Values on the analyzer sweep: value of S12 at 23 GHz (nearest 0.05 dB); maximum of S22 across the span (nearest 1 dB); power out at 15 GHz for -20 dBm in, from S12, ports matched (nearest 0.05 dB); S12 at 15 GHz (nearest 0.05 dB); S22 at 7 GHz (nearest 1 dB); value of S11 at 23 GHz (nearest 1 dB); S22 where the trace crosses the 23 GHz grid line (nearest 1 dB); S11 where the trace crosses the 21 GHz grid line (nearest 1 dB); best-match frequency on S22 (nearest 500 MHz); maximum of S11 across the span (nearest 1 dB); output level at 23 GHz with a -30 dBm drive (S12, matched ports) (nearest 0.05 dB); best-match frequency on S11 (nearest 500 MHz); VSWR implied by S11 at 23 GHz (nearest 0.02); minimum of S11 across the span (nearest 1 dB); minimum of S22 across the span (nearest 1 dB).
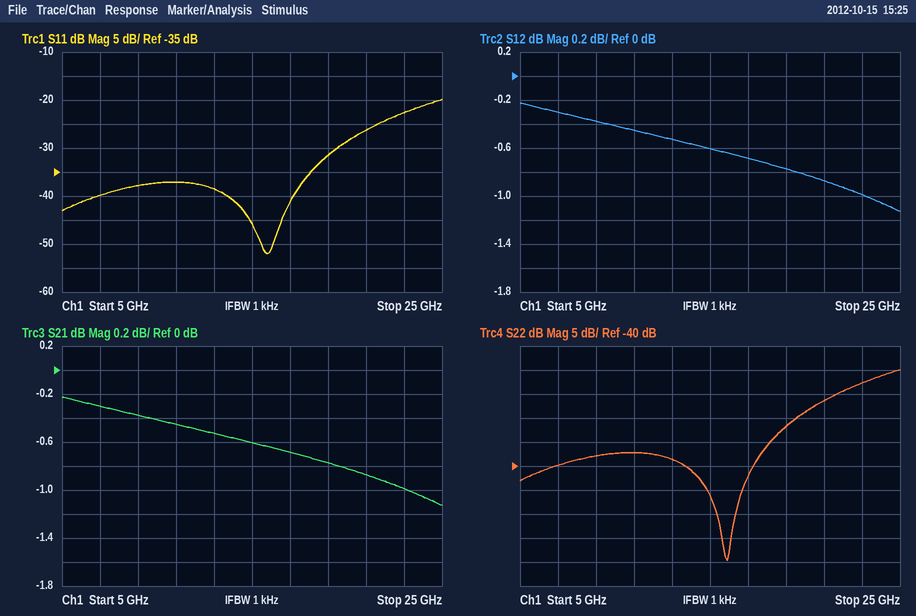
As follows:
-1.00 dB
-20 dB
-20.60 dBm
-0.60 dB
-40 dB
-23 dB
-23 dB
-26 dB
16.0 GHz
-20 dB
-31.00 dBm
16.0 GHz
1.16
-52 dB
-60 dB
